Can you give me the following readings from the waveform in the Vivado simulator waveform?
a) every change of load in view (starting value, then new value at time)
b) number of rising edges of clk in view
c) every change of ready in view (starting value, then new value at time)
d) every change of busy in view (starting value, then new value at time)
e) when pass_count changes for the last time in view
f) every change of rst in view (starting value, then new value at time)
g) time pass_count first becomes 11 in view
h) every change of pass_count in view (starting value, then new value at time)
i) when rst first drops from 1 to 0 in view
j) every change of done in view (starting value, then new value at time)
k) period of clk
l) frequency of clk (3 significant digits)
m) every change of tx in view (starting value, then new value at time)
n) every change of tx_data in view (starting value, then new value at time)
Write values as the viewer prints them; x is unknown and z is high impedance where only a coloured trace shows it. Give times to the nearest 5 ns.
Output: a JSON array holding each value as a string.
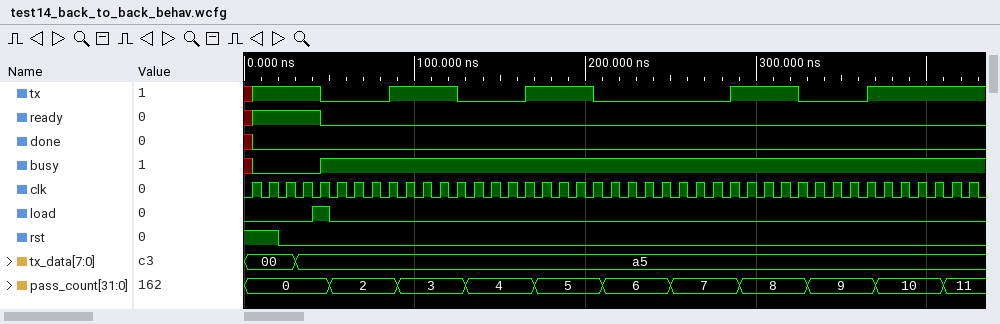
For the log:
["0, 1 at 40 ns, 0 at 50 ns", "43", "x, 1 at 5 ns, 0 at 45 ns", "x, 0 at 5 ns, 1 at 45 ns", "410 ns", "1, 0 at 20 ns", "410 ns", "0, 2 at 50 ns, 3 at 90 ns, 4 at 130 ns, 5 at 170 ns, 6 at 210 ns, 7 at 250 ns, 8 at 290 ns, 9 at 330 ns, 10 at 370 ns, 11 at 410 ns", "20 ns", "x, 0 at 5 ns", "10 ns", "100 MHz", "x, 1 at 5 ns, 0 at 45 ns, 1 at 85 ns, 0 at 125 ns, 1 at 165 ns, 0 at 205 ns, 1 at 285 ns, 0 at 325 ns, 1 at 365 ns", "00, a5 at 30 ns"]
